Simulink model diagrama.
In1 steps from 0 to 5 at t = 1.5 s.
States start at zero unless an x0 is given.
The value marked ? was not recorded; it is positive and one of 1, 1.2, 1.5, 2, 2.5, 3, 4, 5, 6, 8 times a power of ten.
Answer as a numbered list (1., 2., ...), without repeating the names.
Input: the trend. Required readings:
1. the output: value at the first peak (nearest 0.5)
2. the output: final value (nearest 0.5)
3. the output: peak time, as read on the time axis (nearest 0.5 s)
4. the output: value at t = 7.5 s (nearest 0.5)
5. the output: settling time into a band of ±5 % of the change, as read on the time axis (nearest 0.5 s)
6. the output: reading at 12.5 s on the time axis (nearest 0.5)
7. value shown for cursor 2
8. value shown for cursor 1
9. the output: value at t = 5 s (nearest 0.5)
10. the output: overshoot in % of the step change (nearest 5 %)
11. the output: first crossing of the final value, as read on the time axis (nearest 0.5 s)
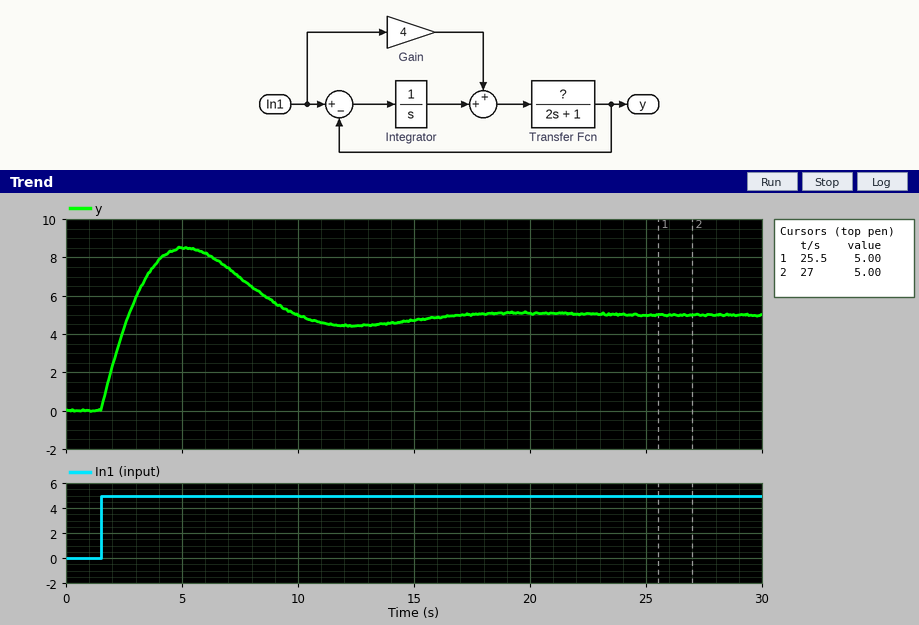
1. 8.5
2. 5.0
3. 5.0 s
4. 7.0
5. 15.0 s
6. 4.5
7. 5.00
8. 5.00
9. 8.5
10. 70 %
11. 2.5 s
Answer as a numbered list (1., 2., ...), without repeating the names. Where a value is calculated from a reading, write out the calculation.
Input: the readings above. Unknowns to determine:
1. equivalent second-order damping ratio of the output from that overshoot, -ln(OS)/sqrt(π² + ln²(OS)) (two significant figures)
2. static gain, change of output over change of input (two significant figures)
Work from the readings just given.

1. ln(0.7) = -0.357; 0.357 / sqrt(9.870 + 0.127) = 0.11
2. (5 - 0) / (5 - 0) = 1.0
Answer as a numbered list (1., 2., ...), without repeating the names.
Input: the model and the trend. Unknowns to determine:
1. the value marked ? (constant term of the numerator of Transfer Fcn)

1. 0.5
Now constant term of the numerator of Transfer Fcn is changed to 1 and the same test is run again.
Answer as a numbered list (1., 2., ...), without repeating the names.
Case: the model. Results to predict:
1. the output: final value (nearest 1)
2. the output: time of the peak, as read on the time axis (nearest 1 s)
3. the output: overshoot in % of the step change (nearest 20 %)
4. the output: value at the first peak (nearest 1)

1. 5
2. 4 s
3. 140 %
4. 12
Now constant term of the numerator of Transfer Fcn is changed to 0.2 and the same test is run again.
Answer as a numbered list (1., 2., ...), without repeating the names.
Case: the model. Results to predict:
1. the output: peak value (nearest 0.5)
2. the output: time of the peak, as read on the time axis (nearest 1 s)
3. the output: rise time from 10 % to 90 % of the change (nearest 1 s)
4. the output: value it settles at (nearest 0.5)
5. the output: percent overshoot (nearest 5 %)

1. 5.5
2. 10 s
3. 3 s
4. 5.0
5. 10 %
